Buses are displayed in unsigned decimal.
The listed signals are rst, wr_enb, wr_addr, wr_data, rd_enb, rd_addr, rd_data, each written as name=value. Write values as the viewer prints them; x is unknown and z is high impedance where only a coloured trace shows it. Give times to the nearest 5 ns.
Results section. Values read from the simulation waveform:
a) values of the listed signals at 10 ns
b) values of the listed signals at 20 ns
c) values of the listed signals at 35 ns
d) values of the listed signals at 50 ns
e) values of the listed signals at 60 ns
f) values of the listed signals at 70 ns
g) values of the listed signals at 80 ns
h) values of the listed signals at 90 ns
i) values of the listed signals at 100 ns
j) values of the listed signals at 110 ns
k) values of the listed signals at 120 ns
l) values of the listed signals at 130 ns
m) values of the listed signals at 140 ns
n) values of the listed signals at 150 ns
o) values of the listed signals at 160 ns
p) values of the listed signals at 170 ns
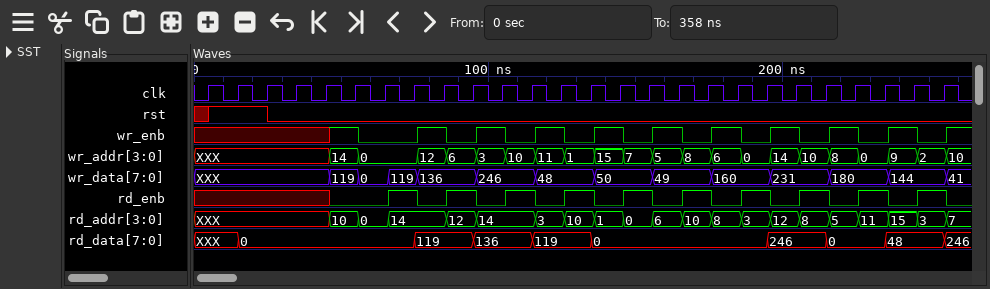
rst=1, wr_enb=x, wr_addr=XXX, wr_data=XXX, rd_enb=x, rd_addr=XXX, rd_data=XXX
rst=1, wr_enb=x, wr_addr=XXX, wr_data=XXX, rd_enb=x, rd_addr=XXX, rd_data=0
rst=0, wr_enb=x, wr_addr=XXX, wr_data=XXX, rd_enb=x, rd_addr=XXX, rd_data=0
rst=0, wr_enb=1, wr_addr=14, wr_data=119, rd_enb=0, rd_addr=10, rd_data=0
rst=0, wr_enb=0, wr_addr=0, wr_data=0, rd_enb=0, rd_addr=0, rd_data=0
rst=0, wr_enb=0, wr_addr=0, wr_data=119, rd_enb=1, rd_addr=14, rd_data=0
rst=0, wr_enb=1, wr_addr=12, wr_data=136, rd_enb=0, rd_addr=14, rd_data=119
rst=0, wr_enb=0, wr_addr=6, wr_data=136, rd_enb=1, rd_addr=12, rd_data=119
rst=0, wr_enb=1, wr_addr=3, wr_data=246, rd_enb=0, rd_addr=14, rd_data=136
rst=0, wr_enb=0, wr_addr=10, wr_data=246, rd_enb=1, rd_addr=14, rd_data=136
rst=0, wr_enb=1, wr_addr=11, wr_data=48, rd_enb=0, rd_addr=3, rd_data=119
rst=0, wr_enb=0, wr_addr=1, wr_data=48, rd_enb=1, rd_addr=10, rd_data=119
rst=0, wr_enb=1, wr_addr=15, wr_data=50, rd_enb=0, rd_addr=1, rd_data=0
rst=0, wr_enb=0, wr_addr=7, wr_data=50, rd_enb=1, rd_addr=0, rd_data=0
rst=0, wr_enb=1, wr_addr=5, wr_data=49, rd_enb=0, rd_addr=6, rd_data=0
rst=0, wr_enb=0, wr_addr=8, wr_data=49, rd_enb=1, rd_addr=10, rd_data=0
